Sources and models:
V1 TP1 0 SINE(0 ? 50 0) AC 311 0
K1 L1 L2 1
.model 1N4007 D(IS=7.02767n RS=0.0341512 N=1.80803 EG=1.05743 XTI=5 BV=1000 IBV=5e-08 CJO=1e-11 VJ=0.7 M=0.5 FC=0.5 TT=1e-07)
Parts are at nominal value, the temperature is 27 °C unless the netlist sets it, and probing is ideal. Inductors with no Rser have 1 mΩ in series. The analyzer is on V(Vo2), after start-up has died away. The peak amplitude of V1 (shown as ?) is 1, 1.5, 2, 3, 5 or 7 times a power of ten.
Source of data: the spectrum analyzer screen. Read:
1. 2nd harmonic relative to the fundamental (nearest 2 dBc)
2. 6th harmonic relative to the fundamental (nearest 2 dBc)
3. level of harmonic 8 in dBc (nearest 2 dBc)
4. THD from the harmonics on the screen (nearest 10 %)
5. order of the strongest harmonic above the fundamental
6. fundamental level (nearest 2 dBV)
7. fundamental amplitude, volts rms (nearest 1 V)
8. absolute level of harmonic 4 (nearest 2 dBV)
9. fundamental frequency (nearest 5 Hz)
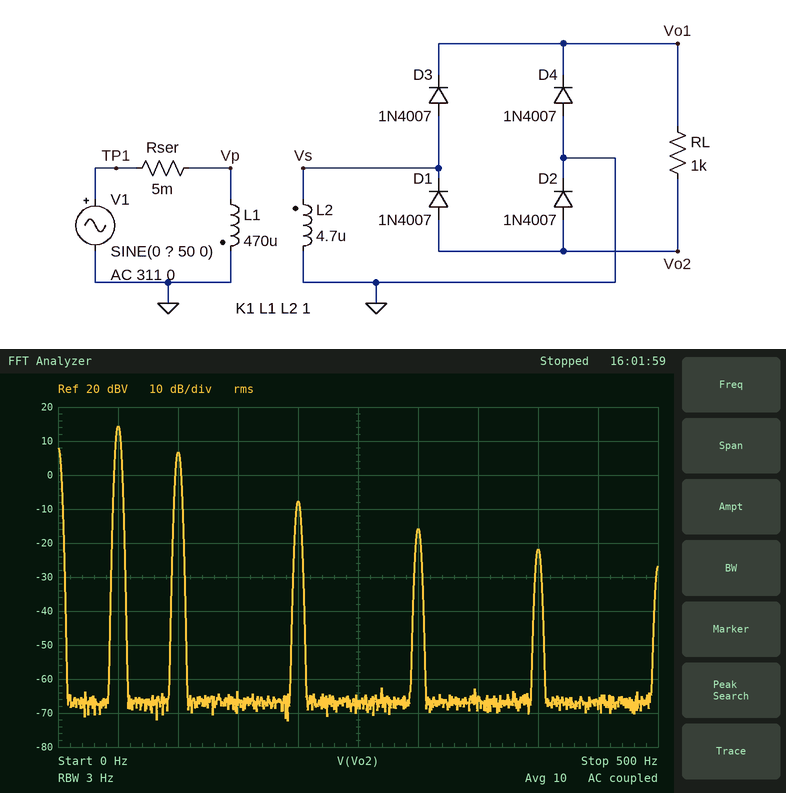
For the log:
-8 dBc
-30 dBc
-36 dBc
40 %
2
14 dBV
5 V
-8 dBV
50 Hz
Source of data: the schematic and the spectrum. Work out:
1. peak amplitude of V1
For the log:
150 V
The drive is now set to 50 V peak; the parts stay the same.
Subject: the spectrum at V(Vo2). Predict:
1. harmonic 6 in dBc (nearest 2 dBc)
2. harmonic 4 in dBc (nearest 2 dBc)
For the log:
-40 dBc
-26 dBc
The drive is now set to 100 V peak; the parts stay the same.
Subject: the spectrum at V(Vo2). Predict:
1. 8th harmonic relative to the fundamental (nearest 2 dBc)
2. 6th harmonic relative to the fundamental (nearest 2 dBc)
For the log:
-38 dBc
-32 dBc
